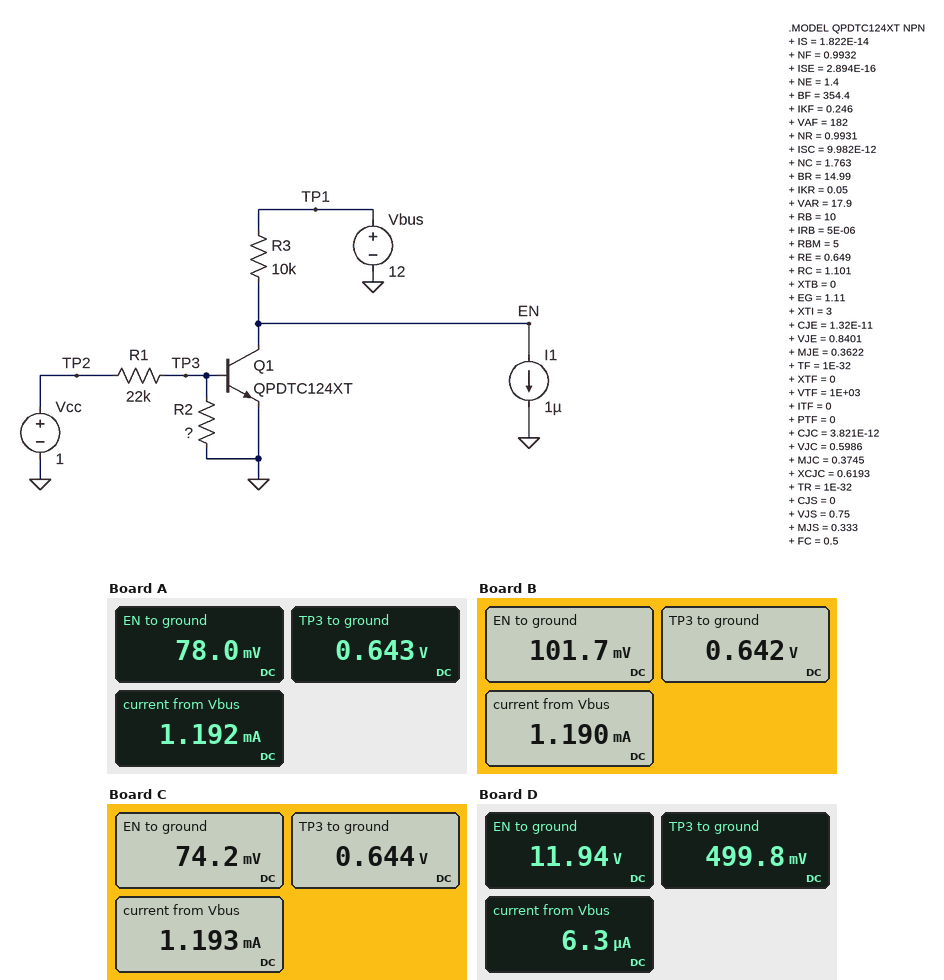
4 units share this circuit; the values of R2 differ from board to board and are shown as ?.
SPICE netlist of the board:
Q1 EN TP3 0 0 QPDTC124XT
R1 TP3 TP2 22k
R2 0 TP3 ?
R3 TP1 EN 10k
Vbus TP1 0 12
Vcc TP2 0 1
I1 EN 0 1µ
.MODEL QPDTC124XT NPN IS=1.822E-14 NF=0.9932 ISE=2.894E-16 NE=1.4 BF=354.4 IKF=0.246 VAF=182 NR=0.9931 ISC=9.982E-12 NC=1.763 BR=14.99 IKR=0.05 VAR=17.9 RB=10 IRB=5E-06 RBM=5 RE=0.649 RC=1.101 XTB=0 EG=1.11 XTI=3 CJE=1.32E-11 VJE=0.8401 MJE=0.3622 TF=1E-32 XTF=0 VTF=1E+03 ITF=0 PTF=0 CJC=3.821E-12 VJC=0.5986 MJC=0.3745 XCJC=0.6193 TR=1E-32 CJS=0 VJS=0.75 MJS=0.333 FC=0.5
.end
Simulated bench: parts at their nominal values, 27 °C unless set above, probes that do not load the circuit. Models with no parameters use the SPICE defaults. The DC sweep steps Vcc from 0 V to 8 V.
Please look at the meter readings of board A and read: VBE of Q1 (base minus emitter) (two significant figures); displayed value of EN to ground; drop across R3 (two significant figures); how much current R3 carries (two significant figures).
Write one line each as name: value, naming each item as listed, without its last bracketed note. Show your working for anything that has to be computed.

VBE of Q1 (base minus emitter): 643 mV = 640 mV
displayed value of EN to ground: 78.0 mV
drop across R3: 12 V - 78 mV = 12 V
how much current R3 carries: (12 V - 78 mV) / 10 kΩ = 1.2 mA
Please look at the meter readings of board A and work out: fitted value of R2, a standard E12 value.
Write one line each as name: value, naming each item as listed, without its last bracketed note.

fitted value of R2, a standard E12 value: 120 kΩ
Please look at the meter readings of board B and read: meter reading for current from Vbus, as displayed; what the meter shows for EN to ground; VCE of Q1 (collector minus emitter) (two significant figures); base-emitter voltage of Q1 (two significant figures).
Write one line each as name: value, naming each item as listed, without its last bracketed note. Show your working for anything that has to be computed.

meter reading for current from Vbus, as displayed: 1.190 mA
what the meter shows for EN to ground: 101.7 mV
VCE of Q1 (collector minus emitter): 101.7 mV = 100 mV
base-emitter voltage of Q1: 642 mV = 640 mV
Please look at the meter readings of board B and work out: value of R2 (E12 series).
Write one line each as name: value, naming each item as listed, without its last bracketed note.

value of R2: 68 kΩ
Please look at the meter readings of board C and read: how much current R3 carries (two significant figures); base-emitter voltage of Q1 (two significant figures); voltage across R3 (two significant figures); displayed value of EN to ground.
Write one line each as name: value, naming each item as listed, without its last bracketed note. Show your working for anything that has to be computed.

how much current R3 carries: (12 V - 74.2 mV) / 10 kΩ = 1.2 mA
base-emitter voltage of Q1: 644 mV = 640 mV
voltage across R3: 12 V - 74.2 mV = 12 V
displayed value of EN to ground: 74.2 mV
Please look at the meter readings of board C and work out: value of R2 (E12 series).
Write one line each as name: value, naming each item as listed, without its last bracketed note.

value of R2: 150 kΩ
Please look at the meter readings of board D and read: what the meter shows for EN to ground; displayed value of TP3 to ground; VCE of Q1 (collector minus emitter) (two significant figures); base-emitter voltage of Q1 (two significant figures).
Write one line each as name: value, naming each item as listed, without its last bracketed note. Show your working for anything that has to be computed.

what the meter shows for EN to ground: 11.94 V
displayed value of TP3 to ground: 499.8 mV
VCE of Q1 (collector minus emitter): 11.94 V = 12 V
base-emitter voltage of Q1: 499.8 mV = 500 mV
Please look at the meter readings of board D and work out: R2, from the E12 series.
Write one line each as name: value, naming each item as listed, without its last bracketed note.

R2, from the E12 series: 22 kΩ
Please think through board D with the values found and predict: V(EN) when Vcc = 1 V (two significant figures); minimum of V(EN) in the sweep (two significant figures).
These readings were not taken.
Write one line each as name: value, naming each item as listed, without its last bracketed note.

V(EN) when Vcc = 1 V: 12 V
minimum of V(EN) in the sweep: 12 mV
